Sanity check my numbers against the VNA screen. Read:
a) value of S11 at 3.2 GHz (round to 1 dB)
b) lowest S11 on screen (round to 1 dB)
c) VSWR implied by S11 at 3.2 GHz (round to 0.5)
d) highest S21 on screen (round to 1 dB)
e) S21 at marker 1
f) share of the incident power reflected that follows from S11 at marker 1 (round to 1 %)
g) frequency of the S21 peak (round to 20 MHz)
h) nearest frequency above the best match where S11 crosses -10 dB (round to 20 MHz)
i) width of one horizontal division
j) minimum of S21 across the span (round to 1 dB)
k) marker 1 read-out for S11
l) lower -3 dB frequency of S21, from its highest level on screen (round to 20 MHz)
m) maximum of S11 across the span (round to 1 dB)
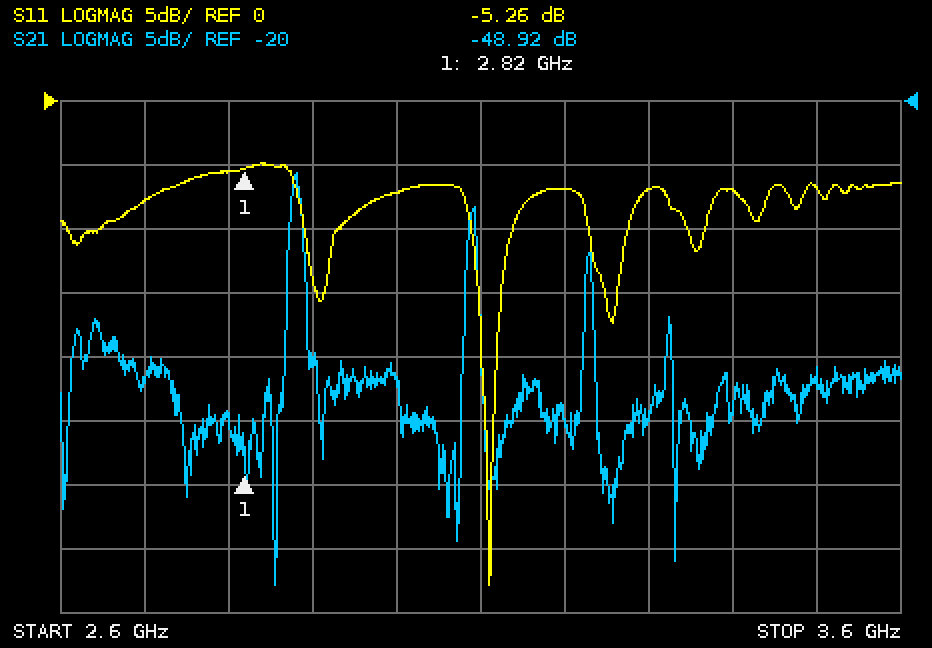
-7 dB
-38 dB
2.5
-26 dB
-48.92 dB
30 %
2.88 GHz
3.14 GHz
100 MHz
-58 dB
-5.26 dB
2.88 GHz
-5 dB
